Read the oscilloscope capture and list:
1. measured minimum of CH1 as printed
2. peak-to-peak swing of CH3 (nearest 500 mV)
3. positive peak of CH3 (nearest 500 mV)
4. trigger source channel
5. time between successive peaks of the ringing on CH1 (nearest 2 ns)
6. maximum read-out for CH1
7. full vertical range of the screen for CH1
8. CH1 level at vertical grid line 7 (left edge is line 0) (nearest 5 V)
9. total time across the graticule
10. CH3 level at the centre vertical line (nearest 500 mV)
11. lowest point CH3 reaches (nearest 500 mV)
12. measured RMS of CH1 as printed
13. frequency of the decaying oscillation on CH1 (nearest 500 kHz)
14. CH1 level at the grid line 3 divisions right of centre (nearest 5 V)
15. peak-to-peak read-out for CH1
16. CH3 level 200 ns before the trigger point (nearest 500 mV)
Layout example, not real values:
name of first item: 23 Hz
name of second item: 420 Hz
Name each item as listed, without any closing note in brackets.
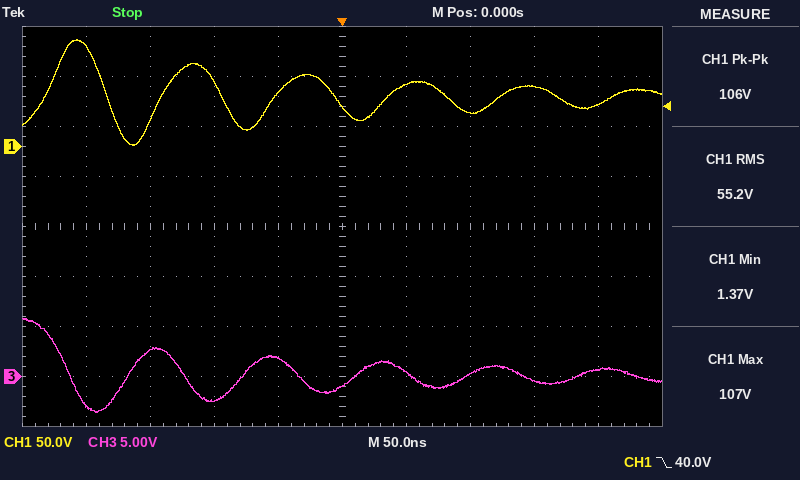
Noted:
measured minimum of CH1 as printed: 1.37 V
peak-to-peak swing of CH3: 9.5 V
positive peak of CH3: 6.0 V
trigger source channel: CH1
time between successive peaks of the ringing on CH1: 88 ns
maximum read-out for CH1: 107 V
full vertical range of the screen for CH1: 400 V
CH1 level at vertical grid line 7 (left edge is line 0): 35 V
total time across the graticule: 500 ns
CH3 level at the centre vertical line: -1.0 V
lowest point CH3 reaches: -3.5 V
measured RMS of CH1 as printed: 55.2 V
frequency of the decaying oscillation on CH1: 11.5 MHz
CH1 level at the grid line 3 divisions right of centre: 60 V
peak-to-peak read-out for CH1: 106 V
CH3 level 200 ns before the trigger point: -3.0 V
